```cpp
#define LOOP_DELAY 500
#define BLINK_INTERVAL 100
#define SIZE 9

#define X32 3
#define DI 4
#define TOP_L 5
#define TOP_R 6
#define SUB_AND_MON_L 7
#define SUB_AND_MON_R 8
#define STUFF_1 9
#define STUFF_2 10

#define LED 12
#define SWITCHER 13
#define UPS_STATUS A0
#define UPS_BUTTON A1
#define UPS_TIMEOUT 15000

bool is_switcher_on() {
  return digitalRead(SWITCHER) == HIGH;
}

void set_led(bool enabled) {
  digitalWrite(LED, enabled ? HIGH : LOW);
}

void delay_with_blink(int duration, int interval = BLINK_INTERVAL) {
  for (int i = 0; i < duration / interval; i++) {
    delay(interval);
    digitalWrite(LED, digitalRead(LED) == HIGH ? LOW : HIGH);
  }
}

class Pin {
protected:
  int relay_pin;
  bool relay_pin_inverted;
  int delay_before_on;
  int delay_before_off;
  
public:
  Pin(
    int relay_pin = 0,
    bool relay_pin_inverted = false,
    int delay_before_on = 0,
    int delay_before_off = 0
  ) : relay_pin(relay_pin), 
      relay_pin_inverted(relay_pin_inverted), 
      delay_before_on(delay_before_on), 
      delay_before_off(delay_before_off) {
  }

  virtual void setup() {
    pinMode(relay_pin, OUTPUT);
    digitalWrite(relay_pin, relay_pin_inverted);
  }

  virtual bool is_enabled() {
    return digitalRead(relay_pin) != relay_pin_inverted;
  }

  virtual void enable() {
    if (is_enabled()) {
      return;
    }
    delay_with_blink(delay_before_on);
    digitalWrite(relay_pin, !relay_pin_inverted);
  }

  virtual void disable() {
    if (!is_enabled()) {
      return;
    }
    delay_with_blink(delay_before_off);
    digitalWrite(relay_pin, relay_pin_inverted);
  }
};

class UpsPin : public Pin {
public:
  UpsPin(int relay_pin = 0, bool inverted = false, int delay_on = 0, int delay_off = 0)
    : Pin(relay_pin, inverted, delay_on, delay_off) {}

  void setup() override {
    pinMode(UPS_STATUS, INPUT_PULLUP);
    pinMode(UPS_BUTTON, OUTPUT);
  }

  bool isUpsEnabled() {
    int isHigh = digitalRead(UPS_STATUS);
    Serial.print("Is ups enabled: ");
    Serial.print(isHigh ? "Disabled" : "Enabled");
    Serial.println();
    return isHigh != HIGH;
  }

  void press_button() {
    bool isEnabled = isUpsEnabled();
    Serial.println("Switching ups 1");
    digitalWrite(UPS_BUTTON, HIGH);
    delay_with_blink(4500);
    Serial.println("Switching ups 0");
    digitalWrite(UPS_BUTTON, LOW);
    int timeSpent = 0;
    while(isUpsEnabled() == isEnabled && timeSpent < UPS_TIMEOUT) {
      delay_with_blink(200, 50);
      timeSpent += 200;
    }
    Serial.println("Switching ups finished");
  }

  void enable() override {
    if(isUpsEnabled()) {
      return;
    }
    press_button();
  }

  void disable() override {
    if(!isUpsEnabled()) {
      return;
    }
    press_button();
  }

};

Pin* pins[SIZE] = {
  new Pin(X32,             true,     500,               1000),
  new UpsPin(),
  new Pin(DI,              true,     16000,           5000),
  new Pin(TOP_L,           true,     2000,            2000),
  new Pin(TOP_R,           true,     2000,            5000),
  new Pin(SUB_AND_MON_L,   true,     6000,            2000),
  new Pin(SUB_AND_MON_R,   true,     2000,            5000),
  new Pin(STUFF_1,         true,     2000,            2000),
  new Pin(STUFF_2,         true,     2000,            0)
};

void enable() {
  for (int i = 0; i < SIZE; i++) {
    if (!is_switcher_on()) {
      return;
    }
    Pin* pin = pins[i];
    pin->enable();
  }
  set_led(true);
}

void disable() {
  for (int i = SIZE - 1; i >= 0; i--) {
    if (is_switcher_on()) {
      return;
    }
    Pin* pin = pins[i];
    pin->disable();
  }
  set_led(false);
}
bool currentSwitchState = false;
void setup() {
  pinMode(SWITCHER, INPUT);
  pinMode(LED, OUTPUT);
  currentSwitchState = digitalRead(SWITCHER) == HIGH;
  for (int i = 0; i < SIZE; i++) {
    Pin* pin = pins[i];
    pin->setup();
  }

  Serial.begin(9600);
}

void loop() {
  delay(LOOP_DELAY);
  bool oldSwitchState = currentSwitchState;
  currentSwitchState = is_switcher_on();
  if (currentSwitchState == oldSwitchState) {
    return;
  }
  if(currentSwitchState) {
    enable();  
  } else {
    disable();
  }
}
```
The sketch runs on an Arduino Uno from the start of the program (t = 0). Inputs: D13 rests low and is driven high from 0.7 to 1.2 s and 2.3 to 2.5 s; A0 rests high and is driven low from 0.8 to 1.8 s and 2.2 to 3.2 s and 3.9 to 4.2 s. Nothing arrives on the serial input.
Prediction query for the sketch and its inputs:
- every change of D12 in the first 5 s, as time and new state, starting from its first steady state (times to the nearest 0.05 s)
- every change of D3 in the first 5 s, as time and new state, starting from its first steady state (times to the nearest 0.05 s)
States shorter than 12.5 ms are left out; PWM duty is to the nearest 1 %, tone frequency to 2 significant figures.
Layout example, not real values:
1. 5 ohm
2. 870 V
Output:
1. 0 s low; 1.1 s high; 1.2 s low; 1.3 s high; 1.4 s low; 1.5 s high; 2.1 s low; 2.2 s high; 2.3 s low; 2.4 s high; 2.5 s low; 2.6 s high; 2.7 s low; 2.8 s high; 2.9 s low
2. 0 s high; 1.5 s low; 3 s high
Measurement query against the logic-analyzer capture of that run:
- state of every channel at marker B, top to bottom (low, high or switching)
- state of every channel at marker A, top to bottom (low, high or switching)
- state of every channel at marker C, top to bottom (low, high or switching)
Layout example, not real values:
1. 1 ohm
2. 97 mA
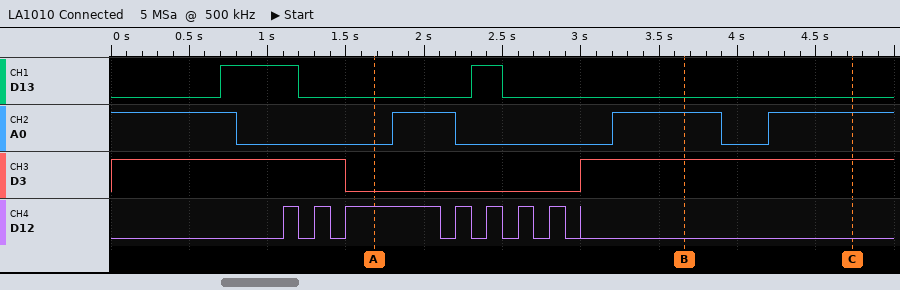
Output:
1. D13 low, A0 high, D3 high, D12 low
2. D13 low, A0 low, D3 low, D12 high
3. D13 low, A0 high, D3 high, D12 low
